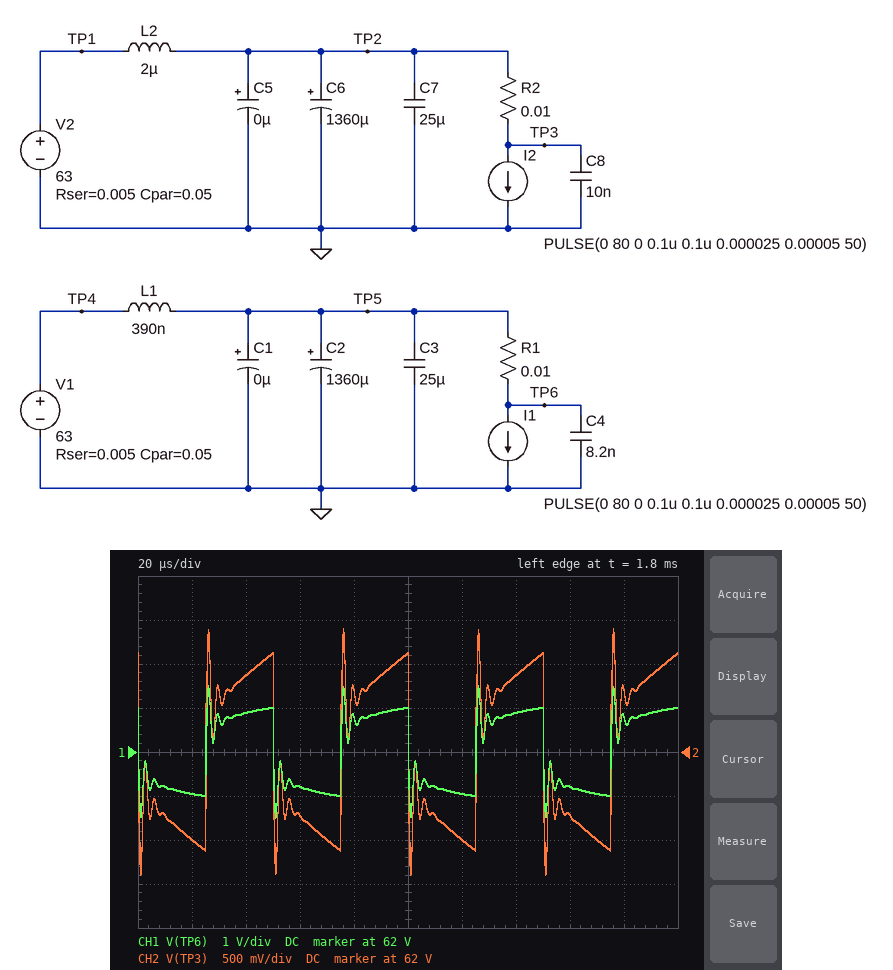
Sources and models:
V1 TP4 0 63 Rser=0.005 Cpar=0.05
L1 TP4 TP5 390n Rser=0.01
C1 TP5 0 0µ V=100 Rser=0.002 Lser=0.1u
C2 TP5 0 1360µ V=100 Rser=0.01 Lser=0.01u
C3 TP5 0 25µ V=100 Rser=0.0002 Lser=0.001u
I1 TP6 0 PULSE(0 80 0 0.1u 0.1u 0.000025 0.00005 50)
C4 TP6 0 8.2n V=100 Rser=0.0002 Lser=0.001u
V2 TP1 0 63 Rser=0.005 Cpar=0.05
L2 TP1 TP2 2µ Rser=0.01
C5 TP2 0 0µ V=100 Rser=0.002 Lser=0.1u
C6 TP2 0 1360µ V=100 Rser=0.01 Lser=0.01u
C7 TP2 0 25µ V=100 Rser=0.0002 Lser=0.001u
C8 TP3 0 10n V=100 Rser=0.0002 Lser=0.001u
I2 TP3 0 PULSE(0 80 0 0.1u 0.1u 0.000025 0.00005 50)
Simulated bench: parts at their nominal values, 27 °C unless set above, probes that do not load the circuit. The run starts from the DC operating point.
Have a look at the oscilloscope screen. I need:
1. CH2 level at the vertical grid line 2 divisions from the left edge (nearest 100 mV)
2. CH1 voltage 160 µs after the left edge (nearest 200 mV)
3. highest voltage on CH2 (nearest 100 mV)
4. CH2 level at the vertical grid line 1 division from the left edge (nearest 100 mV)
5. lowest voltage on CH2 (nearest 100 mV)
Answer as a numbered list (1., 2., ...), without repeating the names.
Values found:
1. 62.9 V
2. 61.2 V
3. 63.4 V
4. 61.0 V
5. 60.6 V
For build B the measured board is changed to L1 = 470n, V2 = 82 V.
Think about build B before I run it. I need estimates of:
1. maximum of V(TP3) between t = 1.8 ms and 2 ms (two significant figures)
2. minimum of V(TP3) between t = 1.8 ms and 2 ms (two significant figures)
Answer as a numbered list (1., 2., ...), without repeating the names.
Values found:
1. 82 V
2. 80 V
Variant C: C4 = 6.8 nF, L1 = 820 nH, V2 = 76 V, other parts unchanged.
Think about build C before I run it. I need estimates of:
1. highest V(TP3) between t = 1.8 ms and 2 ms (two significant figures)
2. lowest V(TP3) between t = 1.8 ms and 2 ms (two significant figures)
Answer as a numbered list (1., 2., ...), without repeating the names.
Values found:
1. 76 V
2. 74 V
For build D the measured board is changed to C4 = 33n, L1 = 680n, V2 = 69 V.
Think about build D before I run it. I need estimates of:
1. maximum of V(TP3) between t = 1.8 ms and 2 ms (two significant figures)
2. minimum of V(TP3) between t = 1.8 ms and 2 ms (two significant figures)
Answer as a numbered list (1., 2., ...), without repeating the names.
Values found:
1. 69 V
2. 67 V
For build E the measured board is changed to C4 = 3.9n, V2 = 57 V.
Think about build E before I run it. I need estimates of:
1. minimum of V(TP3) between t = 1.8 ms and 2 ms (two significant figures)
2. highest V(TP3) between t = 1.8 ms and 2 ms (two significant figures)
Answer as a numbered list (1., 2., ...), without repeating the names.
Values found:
1. 55 V
2. 57 V
